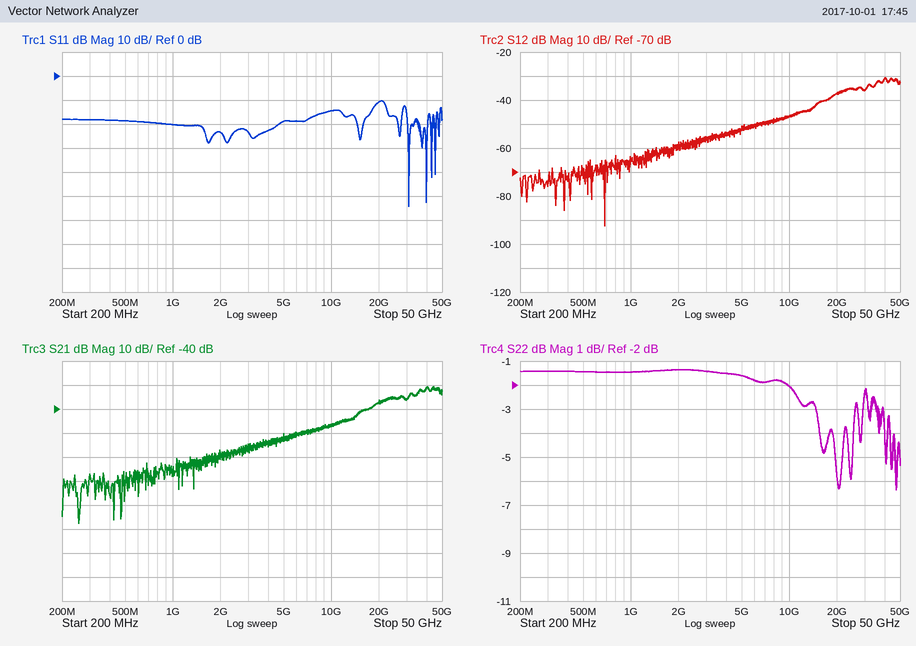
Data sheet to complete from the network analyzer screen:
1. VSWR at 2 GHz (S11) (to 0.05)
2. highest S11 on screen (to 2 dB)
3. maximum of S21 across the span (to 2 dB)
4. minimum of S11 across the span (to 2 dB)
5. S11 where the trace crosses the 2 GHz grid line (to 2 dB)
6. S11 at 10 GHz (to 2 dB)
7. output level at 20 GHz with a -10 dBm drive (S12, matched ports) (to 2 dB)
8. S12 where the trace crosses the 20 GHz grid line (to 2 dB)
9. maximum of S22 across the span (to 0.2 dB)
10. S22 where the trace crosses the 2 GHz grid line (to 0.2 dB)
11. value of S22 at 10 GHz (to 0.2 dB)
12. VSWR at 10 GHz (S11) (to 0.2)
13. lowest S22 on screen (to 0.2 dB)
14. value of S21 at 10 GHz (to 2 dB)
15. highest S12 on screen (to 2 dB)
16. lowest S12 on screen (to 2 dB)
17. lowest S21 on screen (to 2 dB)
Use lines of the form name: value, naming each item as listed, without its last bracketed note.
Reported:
VSWR at 2 GHz (S11): 1.15
highest S11 on screen: -10 dB
maximum of S21 across the span: -30 dB
minimum of S11 across the span: -54 dB
S11 where the trace crosses the 2 GHz grid line: -24 dB
S11 at 10 GHz: -14 dB
output level at 20 GHz with a -10 dBm drive (S12, matched ports): -48 dBm
S12 where the trace crosses the 20 GHz grid line: -38 dB
maximum of S22 across the span: -1.4 dB
S22 where the trace crosses the 2 GHz grid line: -1.4 dB
value of S22 at 10 GHz: -2.0 dB
VSWR at 10 GHz (S11): 1.4
lowest S22 on screen: -6.4 dB
value of S21 at 10 GHz: -46 dB
highest S12 on screen: -30 dB
lowest S12 on screen: -92 dB
lowest S21 on screen: -88 dB
